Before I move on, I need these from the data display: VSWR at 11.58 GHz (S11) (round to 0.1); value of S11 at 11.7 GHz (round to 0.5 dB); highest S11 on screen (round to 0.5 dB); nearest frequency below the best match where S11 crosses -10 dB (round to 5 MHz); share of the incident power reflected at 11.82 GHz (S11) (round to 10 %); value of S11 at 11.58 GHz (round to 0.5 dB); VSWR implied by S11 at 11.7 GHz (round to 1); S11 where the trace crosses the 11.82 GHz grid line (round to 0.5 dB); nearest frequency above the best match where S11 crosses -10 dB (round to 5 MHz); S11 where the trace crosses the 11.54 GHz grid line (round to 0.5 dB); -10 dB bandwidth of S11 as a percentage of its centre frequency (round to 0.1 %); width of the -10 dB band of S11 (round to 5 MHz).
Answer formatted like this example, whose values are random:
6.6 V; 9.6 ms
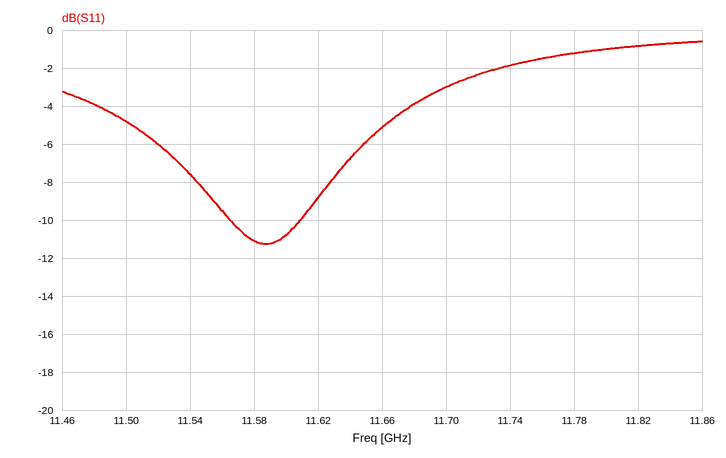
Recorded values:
1.8; -3.0 dB; -0.5 dB; 11.565 GHz; 80 %; -11.0 dB; 6; -1.0 dB; 11.610 GHz; -7.5 dB; 0.4 %; 45 MHz
